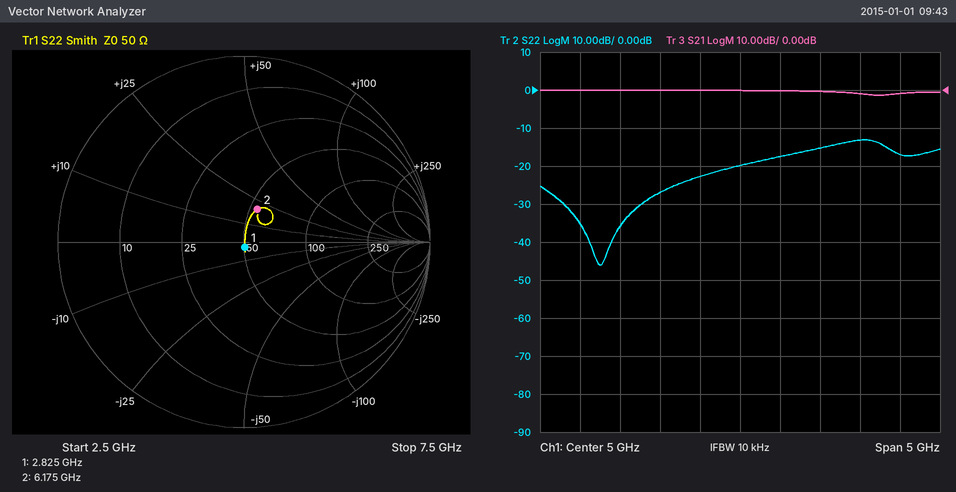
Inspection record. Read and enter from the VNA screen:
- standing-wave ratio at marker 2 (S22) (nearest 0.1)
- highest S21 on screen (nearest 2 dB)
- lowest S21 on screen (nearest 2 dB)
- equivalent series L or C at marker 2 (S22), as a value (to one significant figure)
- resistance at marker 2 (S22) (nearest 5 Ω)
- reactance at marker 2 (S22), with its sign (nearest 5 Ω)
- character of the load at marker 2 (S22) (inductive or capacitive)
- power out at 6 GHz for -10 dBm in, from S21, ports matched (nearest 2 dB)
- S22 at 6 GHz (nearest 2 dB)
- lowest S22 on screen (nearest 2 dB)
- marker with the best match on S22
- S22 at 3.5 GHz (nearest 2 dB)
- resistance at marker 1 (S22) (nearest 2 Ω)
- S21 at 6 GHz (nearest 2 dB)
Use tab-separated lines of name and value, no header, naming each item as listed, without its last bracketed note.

standing-wave ratio at marker 2 (S22)	1.5
highest S21 on screen	0 dB
lowest S21 on screen	-2 dB
equivalent series L or C at marker 2 (S22), as a value	500 pH
resistance at marker 2 (S22)	55 Ω
reactance at marker 2 (S22), with its sign	+20 Ω
character of the load at marker 2 (S22)	inductive
power out at 6 GHz for -10 dBm in, from S21, ports matched	-10 dBm
S22 at 6 GHz	-16 dB
lowest S22 on screen	-46 dB
marker with the best match on S22	marker 1
S22 at 3.5 GHz	-36 dB
resistance at marker 1 (S22)	50 Ω
S21 at 6 GHz	0 dB
